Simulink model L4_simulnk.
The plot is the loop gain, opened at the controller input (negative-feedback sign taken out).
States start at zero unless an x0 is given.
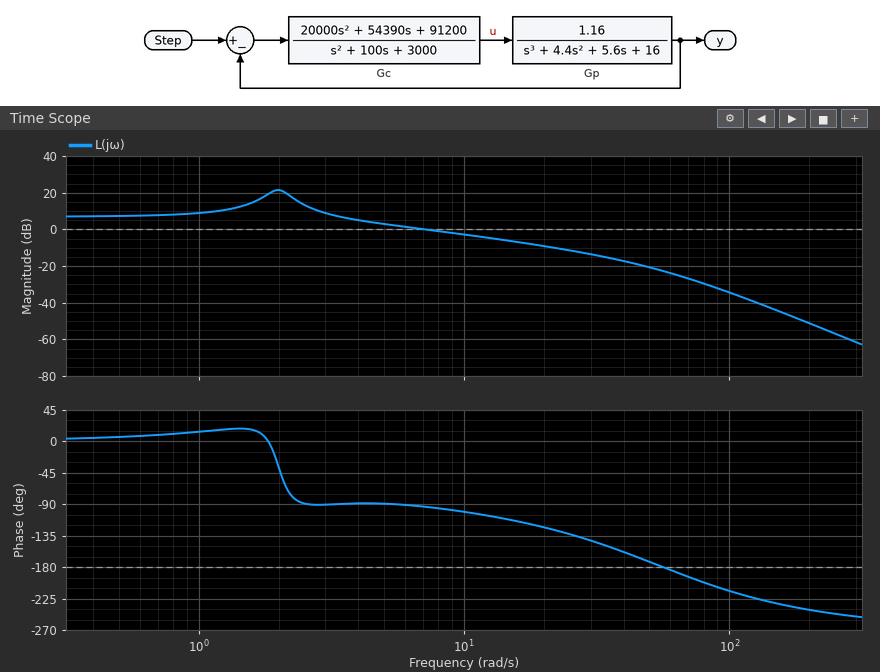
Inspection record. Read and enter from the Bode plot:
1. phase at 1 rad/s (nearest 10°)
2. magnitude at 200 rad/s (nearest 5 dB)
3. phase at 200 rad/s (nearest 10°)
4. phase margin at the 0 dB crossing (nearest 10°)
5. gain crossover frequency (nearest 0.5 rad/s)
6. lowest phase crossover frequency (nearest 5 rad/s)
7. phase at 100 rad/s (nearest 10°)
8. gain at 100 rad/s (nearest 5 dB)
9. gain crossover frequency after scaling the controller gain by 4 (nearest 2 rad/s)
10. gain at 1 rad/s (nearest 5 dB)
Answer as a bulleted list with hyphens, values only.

- 10°
- -50 dB
- -240°
- 90°
- 7.0 rad/s
- 55 rad/s
- -210°
- -35 dB
- 26 rad/s
- 10 dB
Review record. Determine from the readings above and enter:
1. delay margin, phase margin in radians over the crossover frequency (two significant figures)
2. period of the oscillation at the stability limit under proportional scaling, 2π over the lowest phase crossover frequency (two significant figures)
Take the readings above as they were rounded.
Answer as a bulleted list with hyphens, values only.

- 0.22 s
- 0.11 s
